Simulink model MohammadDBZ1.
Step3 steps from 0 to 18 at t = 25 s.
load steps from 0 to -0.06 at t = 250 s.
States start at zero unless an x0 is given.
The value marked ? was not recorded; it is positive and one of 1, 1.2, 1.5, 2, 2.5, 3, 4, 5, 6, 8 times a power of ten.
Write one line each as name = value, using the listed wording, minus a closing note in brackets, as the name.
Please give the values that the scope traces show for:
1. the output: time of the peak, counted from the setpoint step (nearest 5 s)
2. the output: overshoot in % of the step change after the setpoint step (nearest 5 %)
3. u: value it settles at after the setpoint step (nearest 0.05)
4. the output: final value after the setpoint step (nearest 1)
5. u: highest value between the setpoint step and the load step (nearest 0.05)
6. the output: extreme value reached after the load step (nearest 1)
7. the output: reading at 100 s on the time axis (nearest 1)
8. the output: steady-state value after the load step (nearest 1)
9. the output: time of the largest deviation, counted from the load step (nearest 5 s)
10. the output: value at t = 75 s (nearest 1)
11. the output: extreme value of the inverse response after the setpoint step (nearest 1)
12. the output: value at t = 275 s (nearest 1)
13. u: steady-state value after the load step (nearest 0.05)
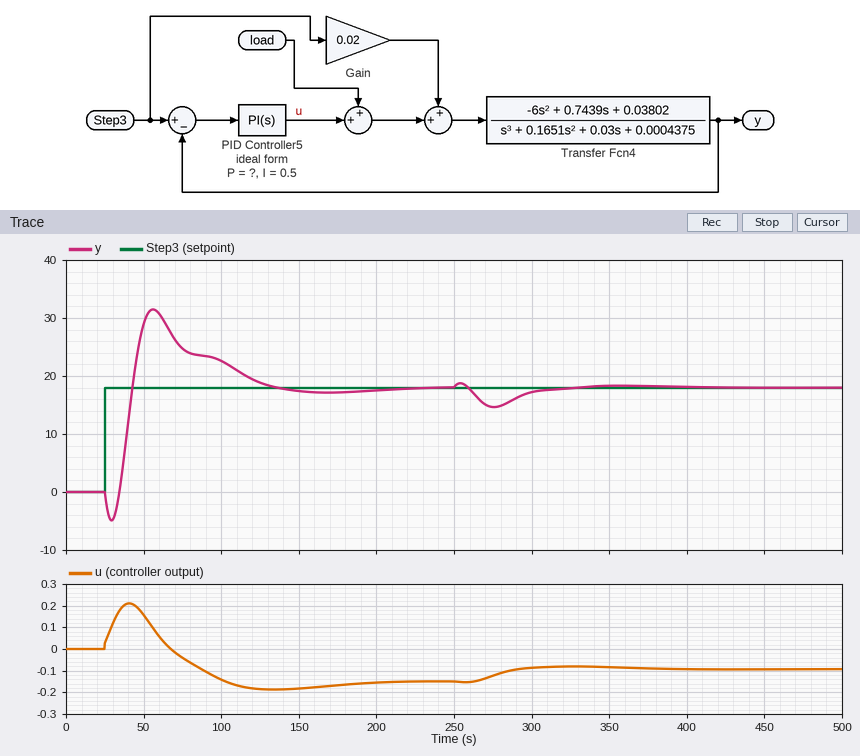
the output: time of the peak, counted from the setpoint step = 30 s
the output: overshoot in % of the step change after the setpoint step = 75 %
u: value it settles at after the setpoint step = -0.15
the output: final value after the setpoint step = 18
u: highest value between the setpoint step and the load step = 0.20
the output: extreme value reached after the load step = 15
the output: reading at 100 s on the time axis = 23
the output: steady-state value after the load step = 18
the output: time of the largest deviation, counted from the load step = 25 s
the output: value at t = 75 s = 25
the output: extreme value of the inverse response after the setpoint step = -5
the output: value at t = 275 s = 15
u: steady-state value after the load step = -0.10
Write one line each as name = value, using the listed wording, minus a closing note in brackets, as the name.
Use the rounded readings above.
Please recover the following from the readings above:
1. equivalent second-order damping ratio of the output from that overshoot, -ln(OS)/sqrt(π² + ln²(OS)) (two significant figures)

equivalent second-order damping ratio of the output from that overshoot, -ln(OS)/sqrt(π² + ln²(OS)) = 0.091
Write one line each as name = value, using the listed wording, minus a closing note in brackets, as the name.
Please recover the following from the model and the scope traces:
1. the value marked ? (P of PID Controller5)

the value marked ? = 0.0015
